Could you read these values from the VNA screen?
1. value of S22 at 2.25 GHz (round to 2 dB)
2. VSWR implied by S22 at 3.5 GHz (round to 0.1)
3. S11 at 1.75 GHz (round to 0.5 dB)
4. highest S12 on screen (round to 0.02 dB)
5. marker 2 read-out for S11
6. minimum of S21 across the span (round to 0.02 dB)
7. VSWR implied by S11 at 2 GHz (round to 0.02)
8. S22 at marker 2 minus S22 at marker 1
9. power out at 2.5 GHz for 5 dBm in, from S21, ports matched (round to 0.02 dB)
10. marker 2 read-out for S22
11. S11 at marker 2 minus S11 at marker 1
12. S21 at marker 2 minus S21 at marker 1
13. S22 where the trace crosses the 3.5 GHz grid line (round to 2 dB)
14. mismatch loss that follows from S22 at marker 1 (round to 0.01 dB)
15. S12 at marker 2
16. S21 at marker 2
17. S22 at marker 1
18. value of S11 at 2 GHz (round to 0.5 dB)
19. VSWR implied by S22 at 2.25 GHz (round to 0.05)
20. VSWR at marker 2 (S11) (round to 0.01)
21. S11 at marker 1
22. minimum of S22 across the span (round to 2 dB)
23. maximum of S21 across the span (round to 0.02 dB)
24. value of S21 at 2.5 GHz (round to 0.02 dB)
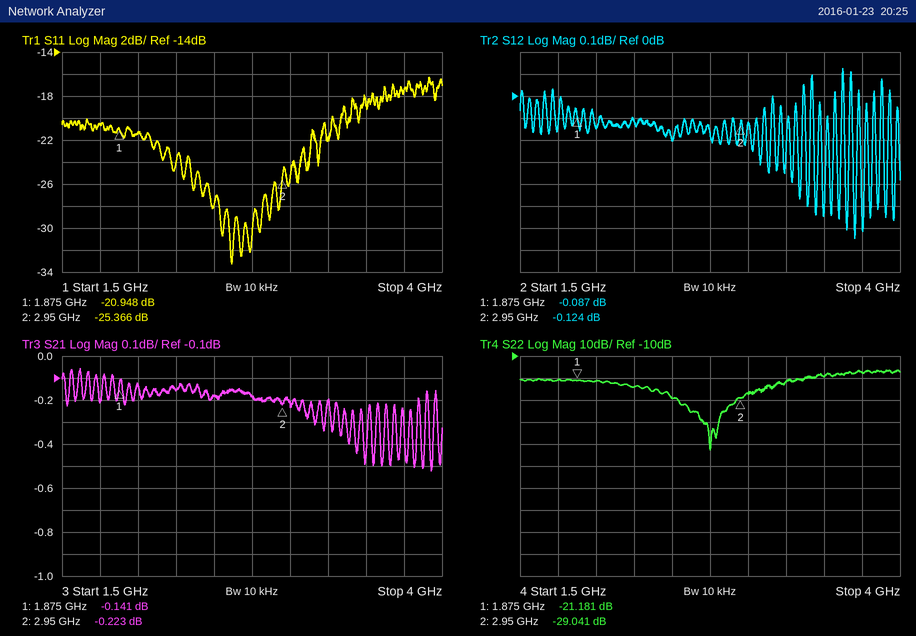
-24 dB
1.2
-20.5 dB
0.12 dB
-25.366 dB
-0.52 dB
1.18
-7.860 dB
4.82 dBm
-29.041 dB
-4.418 dB
-0.082 dB
-20 dB
0.03 dB
-0.124 dB
-0.223 dB
-21.181 dB
-21.5 dB
1.15
1.11
-20.948 dB
-52 dB
-0.06 dB
-0.18 dB
